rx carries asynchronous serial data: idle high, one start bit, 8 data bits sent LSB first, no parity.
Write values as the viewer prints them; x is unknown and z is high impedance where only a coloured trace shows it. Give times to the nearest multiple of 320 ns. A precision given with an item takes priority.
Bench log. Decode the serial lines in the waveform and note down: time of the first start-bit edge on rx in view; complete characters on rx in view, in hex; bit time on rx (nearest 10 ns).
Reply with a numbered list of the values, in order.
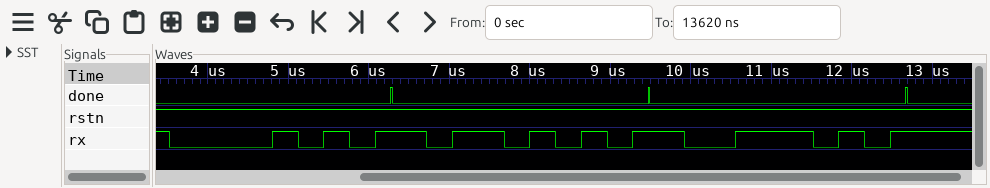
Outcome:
1. 3520 ns
2. A8, AB, AE
3. 320 ns
